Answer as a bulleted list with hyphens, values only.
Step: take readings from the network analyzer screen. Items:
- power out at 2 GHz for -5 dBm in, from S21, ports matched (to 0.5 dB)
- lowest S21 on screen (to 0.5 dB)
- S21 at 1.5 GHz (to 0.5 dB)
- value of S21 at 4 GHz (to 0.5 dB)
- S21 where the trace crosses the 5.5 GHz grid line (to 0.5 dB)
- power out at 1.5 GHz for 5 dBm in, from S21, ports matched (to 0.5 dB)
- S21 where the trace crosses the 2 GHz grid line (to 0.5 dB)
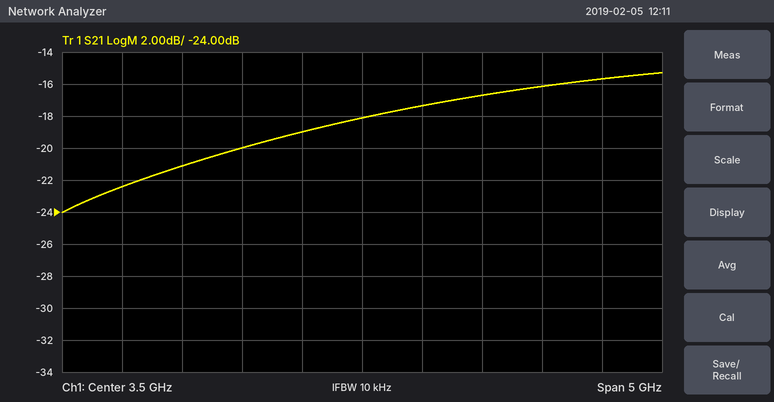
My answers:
- -26.0 dBm
- -24.0 dB
- -22.5 dB
- -17.5 dB
- -15.5 dB
- -17.5 dBm
- -21.0 dB
